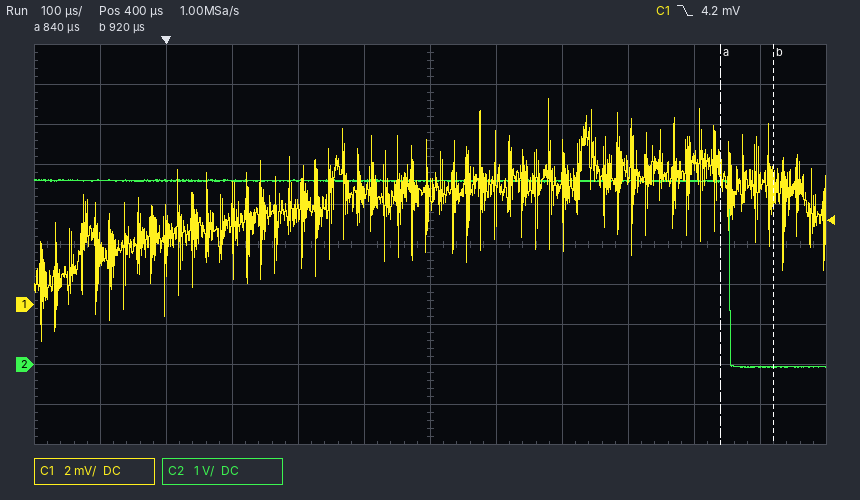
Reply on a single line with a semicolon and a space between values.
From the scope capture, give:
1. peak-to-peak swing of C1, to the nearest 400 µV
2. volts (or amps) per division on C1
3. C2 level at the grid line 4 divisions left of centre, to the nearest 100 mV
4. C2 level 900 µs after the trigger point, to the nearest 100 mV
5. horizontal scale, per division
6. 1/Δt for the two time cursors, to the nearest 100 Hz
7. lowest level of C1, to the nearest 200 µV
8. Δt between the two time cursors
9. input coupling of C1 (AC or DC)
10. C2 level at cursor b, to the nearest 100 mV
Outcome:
12.0 mV; 2 mV; 4.6 V; -100 mV; 100 µs; 12.5 kHz; -1.8 mV; 80 µs; DC; -100 mV
